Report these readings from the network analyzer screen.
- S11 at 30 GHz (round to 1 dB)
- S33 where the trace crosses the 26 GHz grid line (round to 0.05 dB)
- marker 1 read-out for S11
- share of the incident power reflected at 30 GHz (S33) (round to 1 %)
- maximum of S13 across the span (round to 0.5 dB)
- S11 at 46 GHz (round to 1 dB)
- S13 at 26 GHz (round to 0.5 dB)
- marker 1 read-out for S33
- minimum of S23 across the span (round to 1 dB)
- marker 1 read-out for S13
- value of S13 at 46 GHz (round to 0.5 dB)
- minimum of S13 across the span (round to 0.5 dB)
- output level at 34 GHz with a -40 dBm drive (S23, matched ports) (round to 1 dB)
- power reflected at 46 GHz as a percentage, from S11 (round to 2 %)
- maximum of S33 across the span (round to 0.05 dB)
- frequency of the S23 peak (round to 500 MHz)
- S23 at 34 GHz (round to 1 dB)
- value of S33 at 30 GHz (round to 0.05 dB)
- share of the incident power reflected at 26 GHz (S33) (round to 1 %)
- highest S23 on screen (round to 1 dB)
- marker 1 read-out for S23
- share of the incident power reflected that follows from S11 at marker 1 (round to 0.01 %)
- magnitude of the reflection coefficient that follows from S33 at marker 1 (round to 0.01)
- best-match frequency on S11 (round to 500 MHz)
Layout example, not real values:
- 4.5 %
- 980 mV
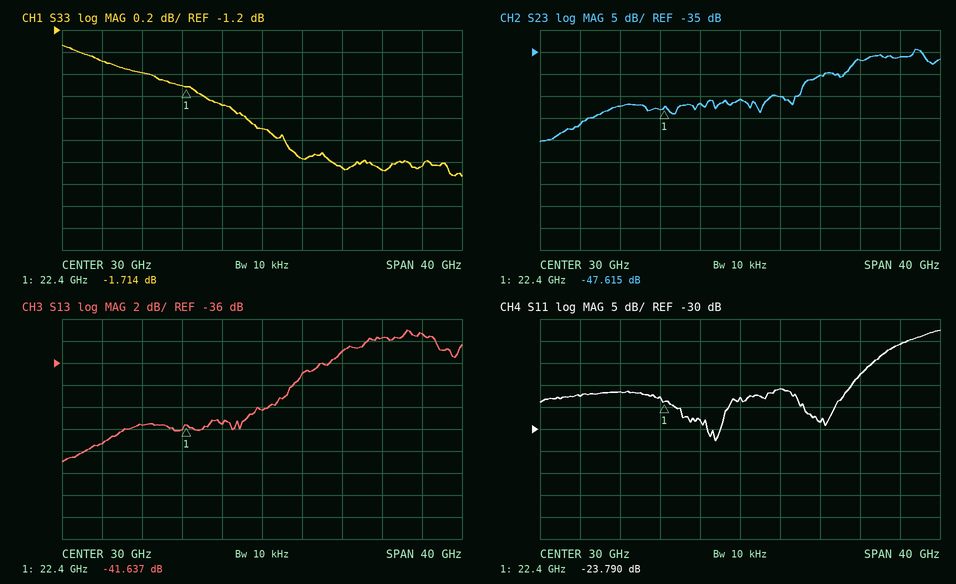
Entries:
- -23 dB
- -1.90 dB
- -23.790 dB
- 62 %
- -33.0 dB
- -11 dB
- -41.5 dB
- -1.714 dB
- -55 dB
- -41.637 dB
- -33.5 dB
- -45.0 dB
- -85 dBm
- 8 %
- -1.35 dB
- 47.5 GHz
- -45 dB
- -2.10 dB
- 65 %
- -34 dB
- -47.615 dB
- 0.42 %
- 0.82
- 27.5 GHz
